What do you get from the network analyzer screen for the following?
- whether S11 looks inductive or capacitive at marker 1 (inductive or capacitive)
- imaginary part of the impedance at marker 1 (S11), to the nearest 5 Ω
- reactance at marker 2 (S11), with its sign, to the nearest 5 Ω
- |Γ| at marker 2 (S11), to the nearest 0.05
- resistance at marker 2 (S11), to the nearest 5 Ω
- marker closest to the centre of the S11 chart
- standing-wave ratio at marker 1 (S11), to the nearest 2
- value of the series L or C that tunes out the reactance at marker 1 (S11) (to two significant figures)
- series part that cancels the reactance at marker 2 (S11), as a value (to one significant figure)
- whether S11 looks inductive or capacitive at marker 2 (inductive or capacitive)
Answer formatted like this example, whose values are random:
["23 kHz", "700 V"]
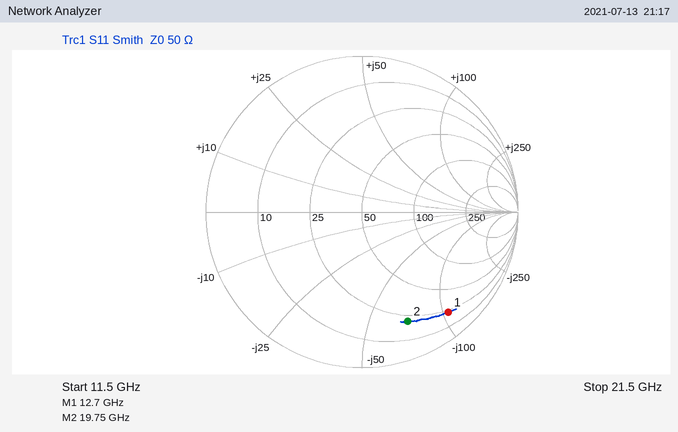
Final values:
["capacitive", "-105 Ω", "-70 Ω", "0.75", "20 Ω", "marker 2", "12", "1.3 nH", "600 pH", "capacitive"]
